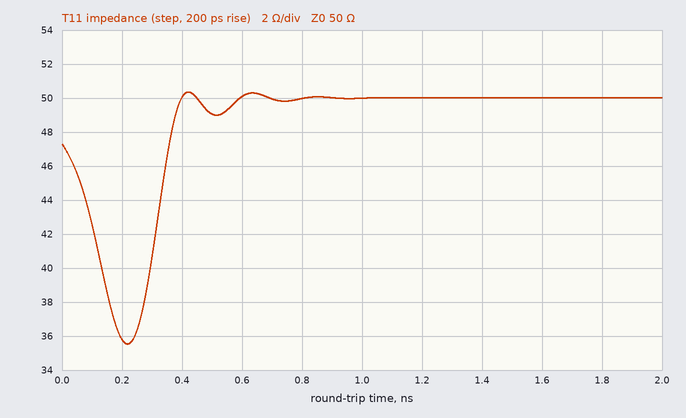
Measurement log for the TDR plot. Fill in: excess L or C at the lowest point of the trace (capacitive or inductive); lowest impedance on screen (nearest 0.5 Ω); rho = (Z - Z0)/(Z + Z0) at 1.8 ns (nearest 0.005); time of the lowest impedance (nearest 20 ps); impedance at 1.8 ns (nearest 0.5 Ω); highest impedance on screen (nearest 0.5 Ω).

capacitive
35.5 Ω
0.000
220 ps
50.0 Ω
50.5 Ω
